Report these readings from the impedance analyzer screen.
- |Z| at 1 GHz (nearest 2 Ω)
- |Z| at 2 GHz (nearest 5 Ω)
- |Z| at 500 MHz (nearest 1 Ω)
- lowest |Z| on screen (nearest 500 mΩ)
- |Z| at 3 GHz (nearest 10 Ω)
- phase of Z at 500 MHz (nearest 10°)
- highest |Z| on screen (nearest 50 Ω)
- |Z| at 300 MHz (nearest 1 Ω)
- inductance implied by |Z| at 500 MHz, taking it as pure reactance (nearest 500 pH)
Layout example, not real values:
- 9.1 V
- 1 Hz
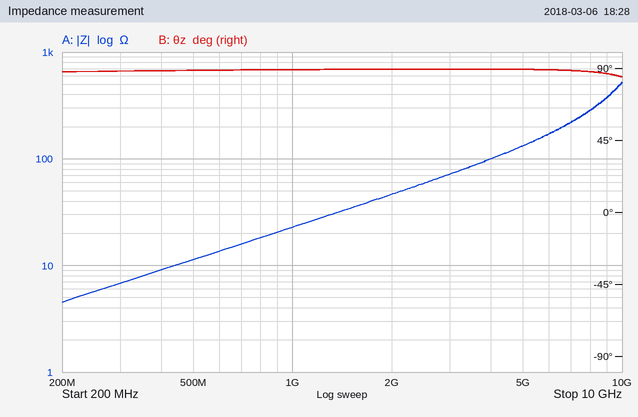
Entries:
- 22 Ω
- 45 Ω
- 11 Ω
- 4.5 Ω
- 70 Ω
- 90°
- 500 Ω
- 7 Ω
- 3.5 nH
